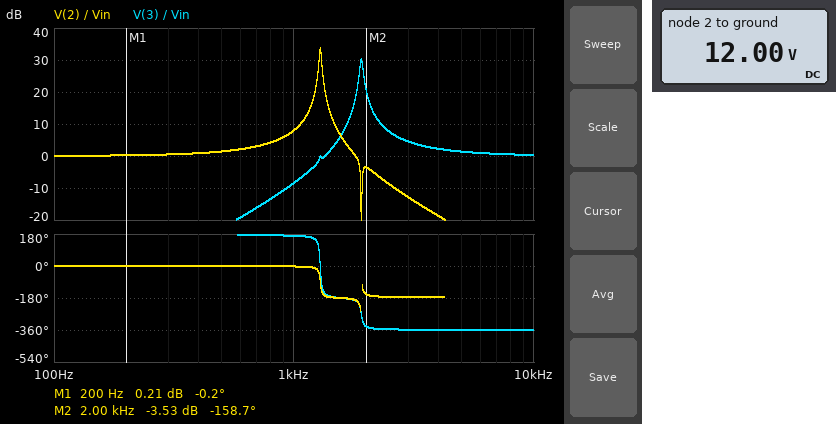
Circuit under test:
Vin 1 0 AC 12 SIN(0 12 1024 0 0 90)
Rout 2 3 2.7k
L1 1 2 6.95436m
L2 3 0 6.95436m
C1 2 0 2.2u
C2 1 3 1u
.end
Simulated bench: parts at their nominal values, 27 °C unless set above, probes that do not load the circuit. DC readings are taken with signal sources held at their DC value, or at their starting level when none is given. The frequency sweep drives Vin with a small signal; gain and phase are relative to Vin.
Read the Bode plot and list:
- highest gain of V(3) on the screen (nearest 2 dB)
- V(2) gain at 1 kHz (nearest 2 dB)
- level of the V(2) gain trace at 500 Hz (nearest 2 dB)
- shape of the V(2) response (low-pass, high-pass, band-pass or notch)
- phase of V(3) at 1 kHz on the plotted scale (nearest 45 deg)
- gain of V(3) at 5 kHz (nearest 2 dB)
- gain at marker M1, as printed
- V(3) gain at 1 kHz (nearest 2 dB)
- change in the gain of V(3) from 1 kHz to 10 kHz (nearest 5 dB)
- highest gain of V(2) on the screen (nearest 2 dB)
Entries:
30 dB
8 dB
2 dB
band-pass
180 deg
2 dB
0.21 dB
-8 dB
10 dB
34 dB
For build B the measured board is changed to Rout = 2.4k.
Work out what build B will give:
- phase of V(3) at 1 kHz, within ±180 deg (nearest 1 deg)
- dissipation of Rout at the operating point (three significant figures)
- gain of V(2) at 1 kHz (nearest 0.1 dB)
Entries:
169 deg
60.0 mW
8.0 dB
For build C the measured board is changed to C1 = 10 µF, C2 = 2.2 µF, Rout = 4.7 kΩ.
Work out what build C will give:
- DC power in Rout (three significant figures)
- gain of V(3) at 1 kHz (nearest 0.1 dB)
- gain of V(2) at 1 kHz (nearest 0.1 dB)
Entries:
30.6 mW
3.7 dB
-4.8 dB
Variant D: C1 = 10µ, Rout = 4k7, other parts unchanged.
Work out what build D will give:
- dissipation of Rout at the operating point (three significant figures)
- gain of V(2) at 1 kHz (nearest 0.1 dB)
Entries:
30.6 mW
-4.8 dB
